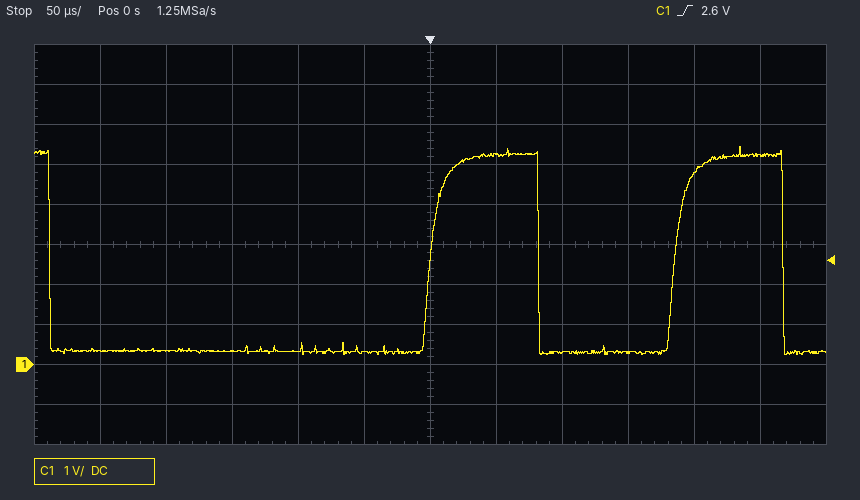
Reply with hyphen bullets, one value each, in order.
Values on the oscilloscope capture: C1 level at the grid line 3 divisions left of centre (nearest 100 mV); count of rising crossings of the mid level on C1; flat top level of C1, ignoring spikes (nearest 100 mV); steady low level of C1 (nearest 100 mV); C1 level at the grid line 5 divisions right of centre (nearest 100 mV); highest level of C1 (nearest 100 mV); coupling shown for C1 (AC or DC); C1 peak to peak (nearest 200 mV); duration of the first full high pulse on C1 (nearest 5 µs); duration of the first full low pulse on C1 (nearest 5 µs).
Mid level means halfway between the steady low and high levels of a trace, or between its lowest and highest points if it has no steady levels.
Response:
- 300 mV
- 2
- 5.2 V
- 300 mV
- 5.2 V
- 5.4 V
- DC
- 5.2 V
- 80 µs
- 290 µs
